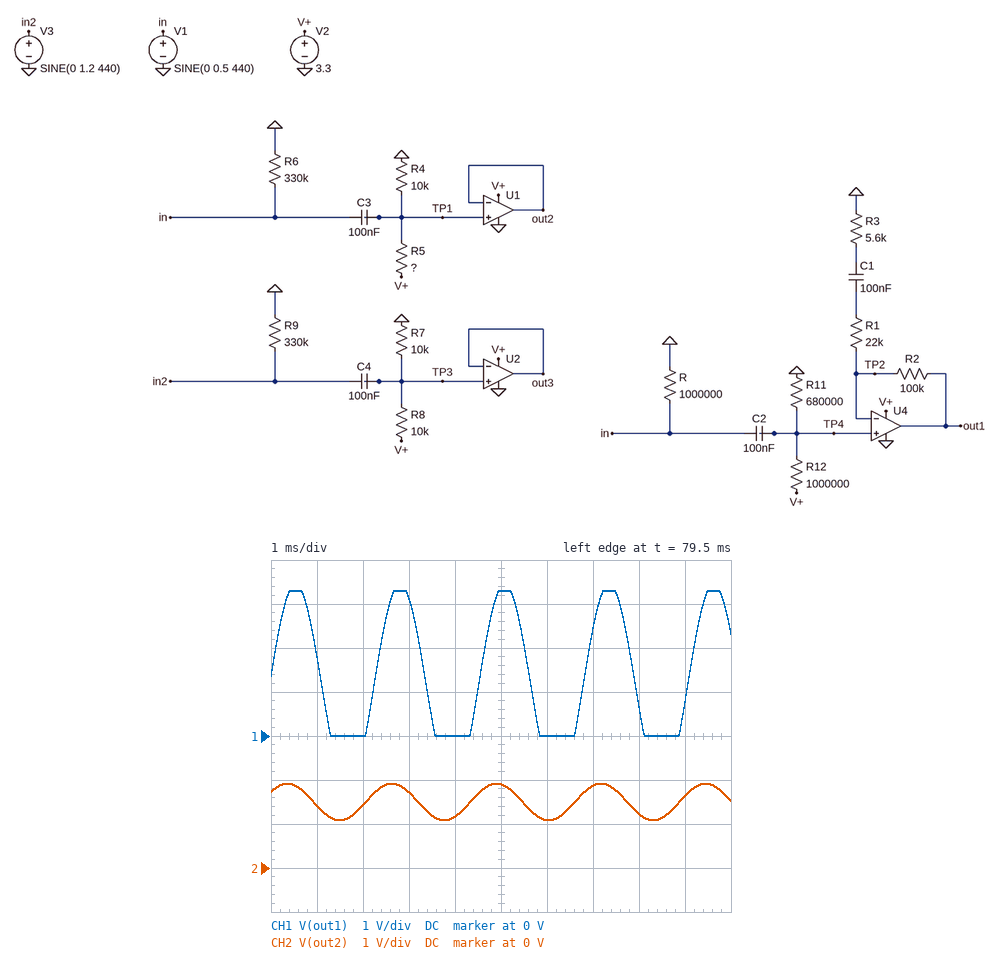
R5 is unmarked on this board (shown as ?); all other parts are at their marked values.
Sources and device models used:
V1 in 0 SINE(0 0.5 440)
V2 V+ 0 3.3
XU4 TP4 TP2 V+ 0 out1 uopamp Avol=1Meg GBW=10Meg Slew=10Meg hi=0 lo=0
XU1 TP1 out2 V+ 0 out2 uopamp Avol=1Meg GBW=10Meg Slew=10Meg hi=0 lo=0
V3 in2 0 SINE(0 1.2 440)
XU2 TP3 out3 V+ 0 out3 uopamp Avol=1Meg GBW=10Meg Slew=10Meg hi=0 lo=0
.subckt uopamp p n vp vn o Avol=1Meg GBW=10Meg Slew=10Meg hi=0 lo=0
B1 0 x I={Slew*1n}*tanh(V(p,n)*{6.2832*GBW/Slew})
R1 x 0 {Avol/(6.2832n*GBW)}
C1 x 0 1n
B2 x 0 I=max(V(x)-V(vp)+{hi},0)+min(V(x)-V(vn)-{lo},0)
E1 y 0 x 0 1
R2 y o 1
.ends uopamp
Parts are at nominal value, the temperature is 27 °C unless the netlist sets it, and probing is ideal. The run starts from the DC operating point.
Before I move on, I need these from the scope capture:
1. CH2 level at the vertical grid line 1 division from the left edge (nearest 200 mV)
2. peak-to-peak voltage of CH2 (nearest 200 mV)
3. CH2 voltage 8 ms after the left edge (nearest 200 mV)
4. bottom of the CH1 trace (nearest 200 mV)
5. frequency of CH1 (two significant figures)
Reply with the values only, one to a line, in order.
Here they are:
1.4 V
800 mV
1.2 V
0 V
440 Hz
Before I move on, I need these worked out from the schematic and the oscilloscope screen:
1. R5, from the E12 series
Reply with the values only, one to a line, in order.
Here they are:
12 kΩ
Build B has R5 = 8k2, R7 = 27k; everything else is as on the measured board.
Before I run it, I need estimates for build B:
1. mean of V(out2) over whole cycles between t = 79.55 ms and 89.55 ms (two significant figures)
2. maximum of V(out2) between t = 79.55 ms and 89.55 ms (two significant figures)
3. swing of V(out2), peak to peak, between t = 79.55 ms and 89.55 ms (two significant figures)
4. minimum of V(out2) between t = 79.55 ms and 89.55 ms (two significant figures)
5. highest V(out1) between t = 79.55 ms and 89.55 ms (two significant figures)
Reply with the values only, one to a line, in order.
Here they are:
1.8 V
2.2 V
780 mV
1.4 V
3.3 V
